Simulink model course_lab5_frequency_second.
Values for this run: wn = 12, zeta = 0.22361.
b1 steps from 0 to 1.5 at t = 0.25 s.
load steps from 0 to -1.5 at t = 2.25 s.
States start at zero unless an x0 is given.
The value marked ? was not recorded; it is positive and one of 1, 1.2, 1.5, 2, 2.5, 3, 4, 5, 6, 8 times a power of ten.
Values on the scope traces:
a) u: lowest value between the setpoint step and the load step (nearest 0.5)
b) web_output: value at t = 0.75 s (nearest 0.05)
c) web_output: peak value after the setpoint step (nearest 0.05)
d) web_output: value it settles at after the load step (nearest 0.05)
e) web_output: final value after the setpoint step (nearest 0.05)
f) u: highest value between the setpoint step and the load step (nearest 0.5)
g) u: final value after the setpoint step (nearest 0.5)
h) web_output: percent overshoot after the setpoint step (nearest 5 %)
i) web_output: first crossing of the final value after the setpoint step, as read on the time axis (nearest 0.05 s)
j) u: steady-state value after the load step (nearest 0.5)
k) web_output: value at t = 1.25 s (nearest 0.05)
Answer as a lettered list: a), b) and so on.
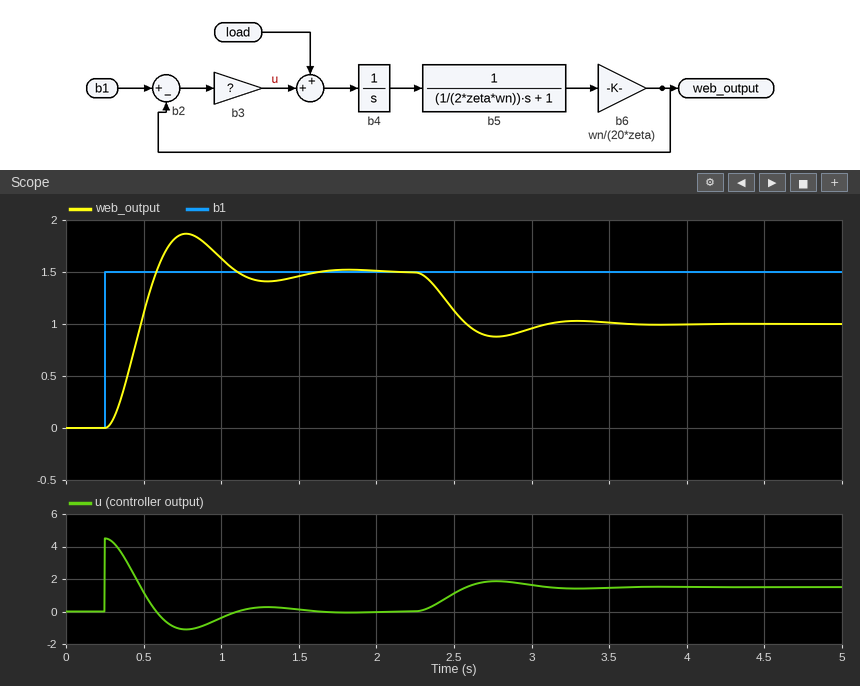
a) -1.0
b) 1.85
c) 1.85
d) 1.00
e) 1.50
f) 4.5
g) 0.0
h) 25 %
i) 0.60 s
j) 1.5
k) 1.40
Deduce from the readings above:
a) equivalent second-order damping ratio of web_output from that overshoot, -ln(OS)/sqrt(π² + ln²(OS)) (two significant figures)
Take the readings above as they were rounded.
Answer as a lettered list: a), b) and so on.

a) 0.40
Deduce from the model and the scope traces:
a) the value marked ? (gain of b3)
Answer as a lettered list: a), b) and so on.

a) 3
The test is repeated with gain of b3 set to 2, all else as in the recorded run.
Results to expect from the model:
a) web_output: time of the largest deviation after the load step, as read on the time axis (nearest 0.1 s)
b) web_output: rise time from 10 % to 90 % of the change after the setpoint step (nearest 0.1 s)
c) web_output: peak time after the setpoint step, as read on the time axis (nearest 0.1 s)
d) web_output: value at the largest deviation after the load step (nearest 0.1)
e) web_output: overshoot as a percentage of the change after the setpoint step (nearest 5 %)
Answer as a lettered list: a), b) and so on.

a) 2.9 s
b) 0.3 s
c) 0.9 s
d) 0.6
e) 15 %
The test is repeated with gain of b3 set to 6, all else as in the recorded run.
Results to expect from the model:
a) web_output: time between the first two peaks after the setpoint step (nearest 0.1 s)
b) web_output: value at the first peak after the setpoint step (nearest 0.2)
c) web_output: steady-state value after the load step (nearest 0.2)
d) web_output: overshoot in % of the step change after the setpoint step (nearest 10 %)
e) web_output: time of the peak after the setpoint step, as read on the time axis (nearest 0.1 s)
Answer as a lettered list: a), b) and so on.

a) 0.7 s
b) 2.0
c) 1.2
d) 40 %
e) 0.6 s
